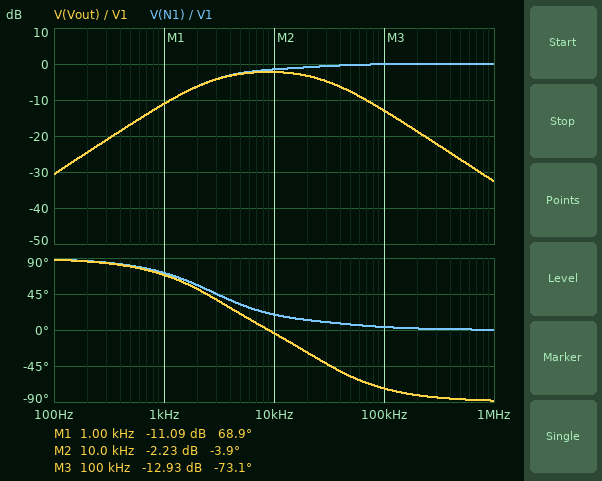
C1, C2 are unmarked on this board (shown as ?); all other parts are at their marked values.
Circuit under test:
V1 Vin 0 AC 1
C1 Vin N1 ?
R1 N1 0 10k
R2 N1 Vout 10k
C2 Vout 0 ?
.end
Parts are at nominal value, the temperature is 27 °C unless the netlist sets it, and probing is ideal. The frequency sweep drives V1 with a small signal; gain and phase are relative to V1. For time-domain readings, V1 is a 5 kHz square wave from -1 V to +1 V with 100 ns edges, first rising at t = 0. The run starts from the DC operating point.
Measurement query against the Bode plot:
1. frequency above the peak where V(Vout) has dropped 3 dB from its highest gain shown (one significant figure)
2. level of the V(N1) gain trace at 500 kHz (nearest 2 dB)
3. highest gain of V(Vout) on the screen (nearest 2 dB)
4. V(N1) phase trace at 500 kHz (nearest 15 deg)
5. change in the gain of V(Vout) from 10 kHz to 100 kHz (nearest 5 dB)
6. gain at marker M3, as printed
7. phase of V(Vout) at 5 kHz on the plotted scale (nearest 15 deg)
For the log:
30 kHz
0 dB
-2 dB
0 deg
-10 dB
-12.93 dB
15 deg
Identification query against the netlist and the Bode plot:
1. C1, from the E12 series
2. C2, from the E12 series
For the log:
4.7 nF
680 pF
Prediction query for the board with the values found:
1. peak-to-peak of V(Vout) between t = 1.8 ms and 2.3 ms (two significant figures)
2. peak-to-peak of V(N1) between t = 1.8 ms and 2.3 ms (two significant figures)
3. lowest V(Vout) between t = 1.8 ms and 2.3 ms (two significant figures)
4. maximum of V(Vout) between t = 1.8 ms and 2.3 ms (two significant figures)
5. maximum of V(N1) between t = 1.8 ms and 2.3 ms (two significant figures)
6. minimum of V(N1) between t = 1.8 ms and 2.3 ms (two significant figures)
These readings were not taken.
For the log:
2.2 V
3.5 V
-1.1 V
1.1 V
1.8 V
-1.8 V
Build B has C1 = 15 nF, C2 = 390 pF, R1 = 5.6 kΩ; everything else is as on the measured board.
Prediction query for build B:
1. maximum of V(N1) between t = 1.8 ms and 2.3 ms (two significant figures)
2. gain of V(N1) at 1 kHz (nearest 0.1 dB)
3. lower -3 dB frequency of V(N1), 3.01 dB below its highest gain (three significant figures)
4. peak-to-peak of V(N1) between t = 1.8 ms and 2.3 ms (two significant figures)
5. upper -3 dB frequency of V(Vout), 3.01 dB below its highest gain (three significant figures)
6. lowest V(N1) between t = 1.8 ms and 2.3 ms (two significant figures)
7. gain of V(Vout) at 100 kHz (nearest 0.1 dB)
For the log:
1.5 V
-6.7 dB
1.95 kHz
3.1 V
45.5 kHz
-1.5 V
-8.5 dB
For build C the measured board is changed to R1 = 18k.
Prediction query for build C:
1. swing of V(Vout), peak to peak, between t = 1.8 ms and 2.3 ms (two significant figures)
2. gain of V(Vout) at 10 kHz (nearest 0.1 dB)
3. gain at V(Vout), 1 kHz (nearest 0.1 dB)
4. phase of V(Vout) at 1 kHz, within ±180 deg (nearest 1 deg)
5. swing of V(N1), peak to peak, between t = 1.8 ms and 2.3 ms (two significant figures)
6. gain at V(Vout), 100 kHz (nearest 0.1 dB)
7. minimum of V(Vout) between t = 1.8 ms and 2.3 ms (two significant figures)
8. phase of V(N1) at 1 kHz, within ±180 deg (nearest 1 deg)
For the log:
2.1 V
-1.9 dB
-6.9 dB
56 deg
3.1 V
-12.9 dB
-1.0 V
59 deg
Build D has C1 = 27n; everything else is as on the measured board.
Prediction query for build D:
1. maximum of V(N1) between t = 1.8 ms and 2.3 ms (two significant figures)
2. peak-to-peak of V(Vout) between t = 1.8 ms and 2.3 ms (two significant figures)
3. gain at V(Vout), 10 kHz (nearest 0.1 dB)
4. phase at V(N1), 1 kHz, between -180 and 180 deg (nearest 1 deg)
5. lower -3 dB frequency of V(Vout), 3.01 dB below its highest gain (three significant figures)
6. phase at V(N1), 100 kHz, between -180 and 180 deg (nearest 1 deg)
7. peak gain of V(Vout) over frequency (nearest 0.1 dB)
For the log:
1.2 V
2.1 V
-0.9 dB
30 deg
549 Hz
1 deg
-0.4 dB
